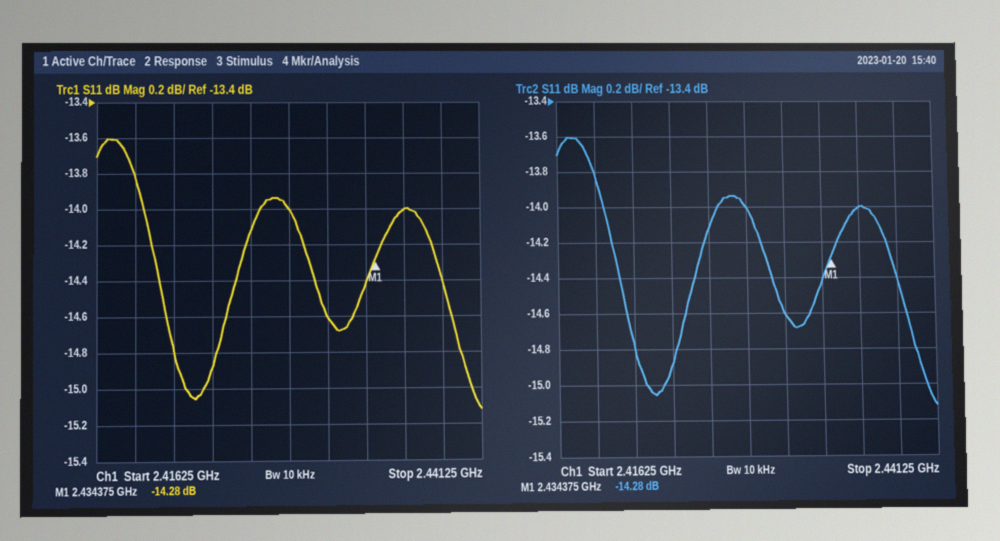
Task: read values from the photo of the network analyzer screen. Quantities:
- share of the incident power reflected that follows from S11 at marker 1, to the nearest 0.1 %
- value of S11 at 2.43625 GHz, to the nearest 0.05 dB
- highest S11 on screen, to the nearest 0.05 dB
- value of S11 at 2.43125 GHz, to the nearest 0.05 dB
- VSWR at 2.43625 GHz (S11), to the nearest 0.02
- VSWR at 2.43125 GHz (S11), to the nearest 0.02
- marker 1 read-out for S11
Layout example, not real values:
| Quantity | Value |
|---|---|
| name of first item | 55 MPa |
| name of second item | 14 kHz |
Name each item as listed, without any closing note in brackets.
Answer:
| Quantity | Value |
|---|---|
| share of the incident power reflected that follows from S11 at marker 1, to the nearest 0.1 % | 3.7 % |
| value of S11 at 2.43625 GHz, to the nearest 0.05 dB | -14.00 dB |
| highest S11 on screen, to the nearest 0.05 dB | -13.60 dB |
| value of S11 at 2.43125 GHz, to the nearest 0.05 dB | -14.60 dB |
| VSWR at 2.43625 GHz (S11), to the nearest 0.02 | 1.50 |
| VSWR at 2.43125 GHz (S11), to the nearest 0.02 | 1.46 |
| marker 1 read-out for S11 | -14.28 dB |
